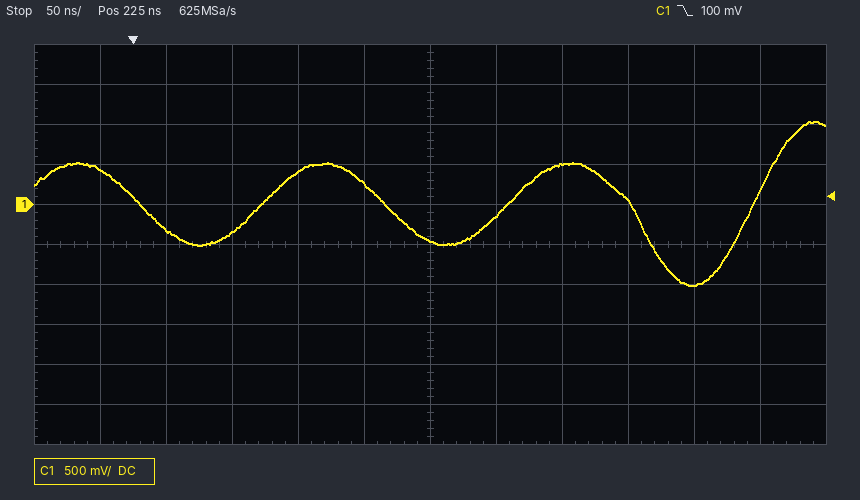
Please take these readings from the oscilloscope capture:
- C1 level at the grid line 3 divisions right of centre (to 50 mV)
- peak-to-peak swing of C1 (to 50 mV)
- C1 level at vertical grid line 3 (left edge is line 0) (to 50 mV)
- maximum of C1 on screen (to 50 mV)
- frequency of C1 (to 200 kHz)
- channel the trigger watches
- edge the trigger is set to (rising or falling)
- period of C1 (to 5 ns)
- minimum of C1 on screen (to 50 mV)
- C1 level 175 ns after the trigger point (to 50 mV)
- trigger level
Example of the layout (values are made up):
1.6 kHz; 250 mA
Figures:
50 mV; 2.05 V; -350 mV; 1.05 V; 5.4 MHz; C1; falling; 185 ns; -1.00 V; 250 mV; 100 mV
